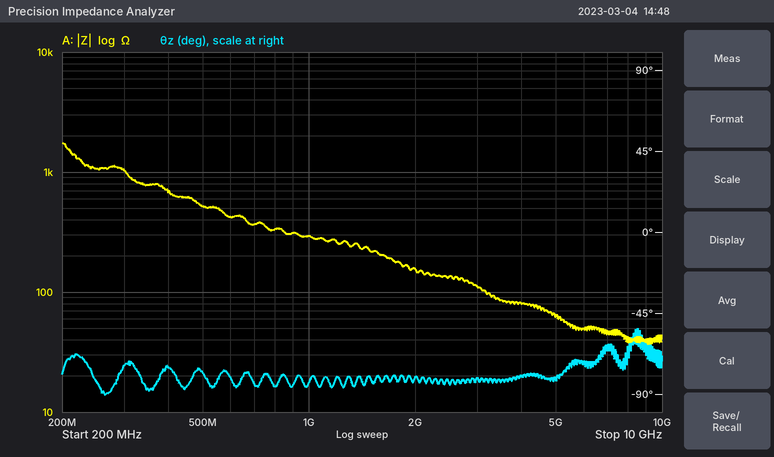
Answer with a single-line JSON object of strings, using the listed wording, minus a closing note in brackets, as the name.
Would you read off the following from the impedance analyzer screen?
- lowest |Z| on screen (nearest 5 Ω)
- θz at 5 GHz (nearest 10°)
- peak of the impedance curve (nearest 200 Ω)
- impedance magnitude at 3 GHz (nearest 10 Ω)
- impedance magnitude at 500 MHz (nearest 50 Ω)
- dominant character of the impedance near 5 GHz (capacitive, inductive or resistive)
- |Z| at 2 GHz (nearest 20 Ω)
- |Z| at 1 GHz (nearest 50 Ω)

{"lowest |Z| on screen": "35 Ω", "θz at 5 GHz": "-80°", "peak of the impedance curve": "1.8 kΩ", "impedance magnitude at 3 GHz": "110 Ω", "impedance magnitude at 500 MHz": "500 Ω", "dominant character of the impedance near 5 GHz": "capacitive", "|Z| at 2 GHz": "160 Ω", "|Z| at 1 GHz": "300 Ω"}
